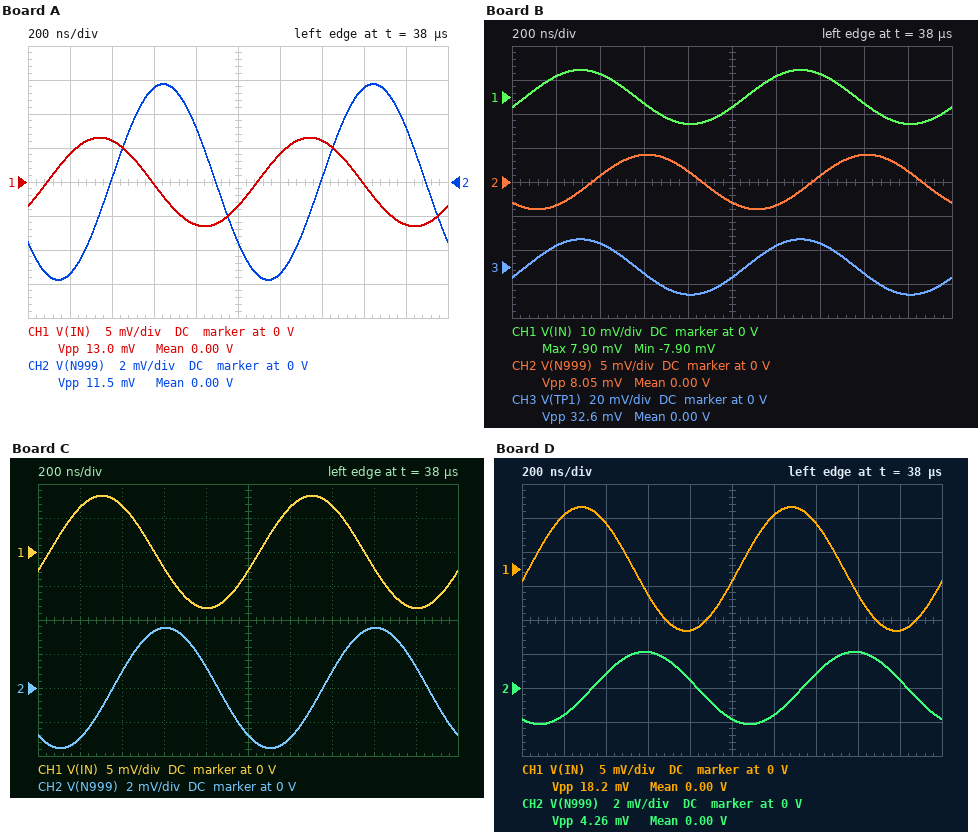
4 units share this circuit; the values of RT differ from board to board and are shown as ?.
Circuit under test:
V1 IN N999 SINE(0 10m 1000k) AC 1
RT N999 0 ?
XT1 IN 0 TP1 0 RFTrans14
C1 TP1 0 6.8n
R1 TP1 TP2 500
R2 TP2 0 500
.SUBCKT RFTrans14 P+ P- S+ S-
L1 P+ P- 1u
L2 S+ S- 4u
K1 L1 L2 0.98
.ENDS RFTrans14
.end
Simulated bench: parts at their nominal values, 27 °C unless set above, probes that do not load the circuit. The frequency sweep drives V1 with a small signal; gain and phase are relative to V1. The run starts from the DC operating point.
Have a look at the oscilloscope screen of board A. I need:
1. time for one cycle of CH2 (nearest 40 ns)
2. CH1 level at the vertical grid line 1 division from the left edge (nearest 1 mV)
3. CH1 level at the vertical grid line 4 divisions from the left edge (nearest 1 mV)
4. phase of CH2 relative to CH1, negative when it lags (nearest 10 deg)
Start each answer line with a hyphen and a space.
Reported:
- 1.00 µs
- 4 mV
- -6 mV
- -110 deg
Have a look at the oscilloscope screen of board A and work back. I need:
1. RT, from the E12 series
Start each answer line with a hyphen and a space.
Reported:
- 68 Ω
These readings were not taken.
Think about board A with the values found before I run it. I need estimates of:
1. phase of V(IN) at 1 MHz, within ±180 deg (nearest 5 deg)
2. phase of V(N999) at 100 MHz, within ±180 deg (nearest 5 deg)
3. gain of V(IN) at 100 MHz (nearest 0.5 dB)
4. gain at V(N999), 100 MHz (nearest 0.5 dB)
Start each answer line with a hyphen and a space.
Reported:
- -35 deg
- 160 deg
- -9.5 dB
- -0.5 dB
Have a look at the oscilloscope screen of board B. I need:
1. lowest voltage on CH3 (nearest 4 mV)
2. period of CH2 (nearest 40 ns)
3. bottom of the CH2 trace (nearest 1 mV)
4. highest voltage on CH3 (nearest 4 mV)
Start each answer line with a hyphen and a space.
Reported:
- -16 mV
- 1.00 µs
- -4 mV
- 16 mV
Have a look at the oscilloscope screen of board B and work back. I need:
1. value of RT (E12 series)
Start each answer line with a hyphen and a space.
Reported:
- 39 Ω
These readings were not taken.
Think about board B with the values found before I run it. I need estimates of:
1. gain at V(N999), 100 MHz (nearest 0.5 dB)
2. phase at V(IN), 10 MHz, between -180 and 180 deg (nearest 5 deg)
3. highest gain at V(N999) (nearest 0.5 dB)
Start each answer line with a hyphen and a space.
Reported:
- -1.5 dB
- 85 deg
- 0 dB
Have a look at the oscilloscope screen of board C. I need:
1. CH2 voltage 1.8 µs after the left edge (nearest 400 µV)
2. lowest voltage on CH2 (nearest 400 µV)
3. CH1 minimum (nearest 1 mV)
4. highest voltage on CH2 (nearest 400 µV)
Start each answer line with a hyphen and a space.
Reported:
- 1.2 mV
- -3.6 mV
- -8 mV
- 3.6 mV
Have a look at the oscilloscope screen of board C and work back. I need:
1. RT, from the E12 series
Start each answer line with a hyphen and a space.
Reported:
- 33 Ω
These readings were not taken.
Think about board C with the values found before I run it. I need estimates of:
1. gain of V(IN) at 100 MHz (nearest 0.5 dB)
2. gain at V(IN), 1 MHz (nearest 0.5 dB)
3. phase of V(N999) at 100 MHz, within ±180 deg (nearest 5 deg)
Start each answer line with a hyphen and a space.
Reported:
- -4.5 dB
- -1.5 dB
- 145 deg
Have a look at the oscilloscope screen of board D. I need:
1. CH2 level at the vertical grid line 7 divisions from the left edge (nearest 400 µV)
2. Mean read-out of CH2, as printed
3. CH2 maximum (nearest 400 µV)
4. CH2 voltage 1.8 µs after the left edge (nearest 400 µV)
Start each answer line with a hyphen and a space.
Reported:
- 800 µV
- 0.00 V
- 2.0 mV
- 400 µV
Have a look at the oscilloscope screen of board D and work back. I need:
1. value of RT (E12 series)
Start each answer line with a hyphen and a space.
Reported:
- 18 Ω
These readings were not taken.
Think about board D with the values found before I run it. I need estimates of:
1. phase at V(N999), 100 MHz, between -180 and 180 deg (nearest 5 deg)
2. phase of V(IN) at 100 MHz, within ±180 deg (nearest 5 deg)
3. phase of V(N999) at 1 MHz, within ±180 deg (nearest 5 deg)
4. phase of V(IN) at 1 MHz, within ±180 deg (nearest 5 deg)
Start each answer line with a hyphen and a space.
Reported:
- 125 deg
- 35 deg
- -120 deg
- -10 deg
